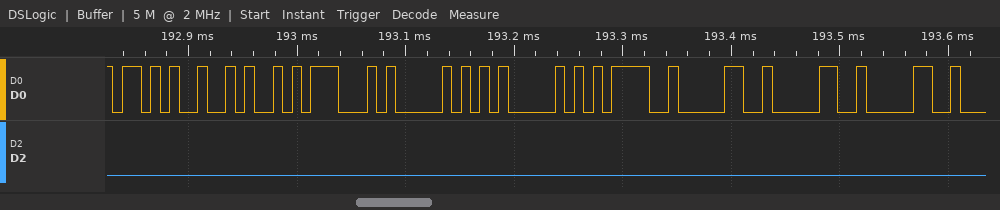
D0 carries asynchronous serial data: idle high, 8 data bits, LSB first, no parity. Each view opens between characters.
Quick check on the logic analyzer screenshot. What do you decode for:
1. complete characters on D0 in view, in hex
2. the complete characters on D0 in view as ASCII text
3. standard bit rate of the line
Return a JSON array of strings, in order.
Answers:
["2B, 4A, 47, 50, 41, 3D, 30, 30, 30", "\"+JGPA=000\"", "115200 baud"]
